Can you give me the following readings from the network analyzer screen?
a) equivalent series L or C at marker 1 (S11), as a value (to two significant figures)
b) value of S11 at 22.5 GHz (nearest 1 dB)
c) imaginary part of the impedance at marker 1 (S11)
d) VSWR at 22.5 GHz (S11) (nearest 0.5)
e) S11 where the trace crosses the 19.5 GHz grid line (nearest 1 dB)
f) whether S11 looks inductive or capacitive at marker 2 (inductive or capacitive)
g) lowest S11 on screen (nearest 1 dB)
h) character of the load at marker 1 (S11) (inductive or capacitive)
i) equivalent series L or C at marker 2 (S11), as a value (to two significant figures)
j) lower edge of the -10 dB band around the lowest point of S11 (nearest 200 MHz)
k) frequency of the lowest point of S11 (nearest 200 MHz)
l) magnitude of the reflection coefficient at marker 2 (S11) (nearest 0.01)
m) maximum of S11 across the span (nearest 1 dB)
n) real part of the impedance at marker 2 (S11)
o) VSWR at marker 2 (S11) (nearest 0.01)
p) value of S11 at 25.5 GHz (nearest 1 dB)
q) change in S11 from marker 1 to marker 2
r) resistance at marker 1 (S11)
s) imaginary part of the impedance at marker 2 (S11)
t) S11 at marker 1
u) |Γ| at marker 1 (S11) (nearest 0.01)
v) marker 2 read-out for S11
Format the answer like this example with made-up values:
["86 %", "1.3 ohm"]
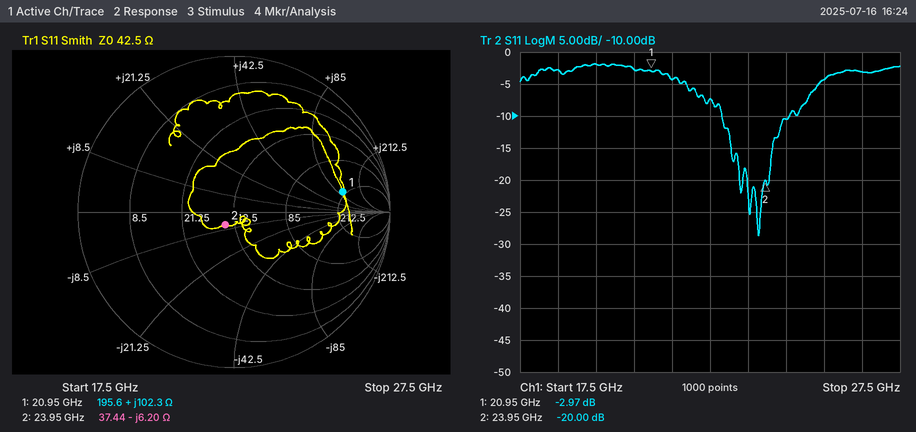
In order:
["780 pH", "-7 dB", "+102.3 Ω", "2.5", "-2 dB", "capacitive", "-29 dB", "inductive", "1.1 pF", "22.8 GHz", "23.8 GHz", "0.10", "-2 dB", "37.44 Ω", "1.22", "-4 dB", "-17.03 dB", "195.6 Ω", "-6.20 Ω", "-2.97 dB", "0.71", "-20.00 dB"]
